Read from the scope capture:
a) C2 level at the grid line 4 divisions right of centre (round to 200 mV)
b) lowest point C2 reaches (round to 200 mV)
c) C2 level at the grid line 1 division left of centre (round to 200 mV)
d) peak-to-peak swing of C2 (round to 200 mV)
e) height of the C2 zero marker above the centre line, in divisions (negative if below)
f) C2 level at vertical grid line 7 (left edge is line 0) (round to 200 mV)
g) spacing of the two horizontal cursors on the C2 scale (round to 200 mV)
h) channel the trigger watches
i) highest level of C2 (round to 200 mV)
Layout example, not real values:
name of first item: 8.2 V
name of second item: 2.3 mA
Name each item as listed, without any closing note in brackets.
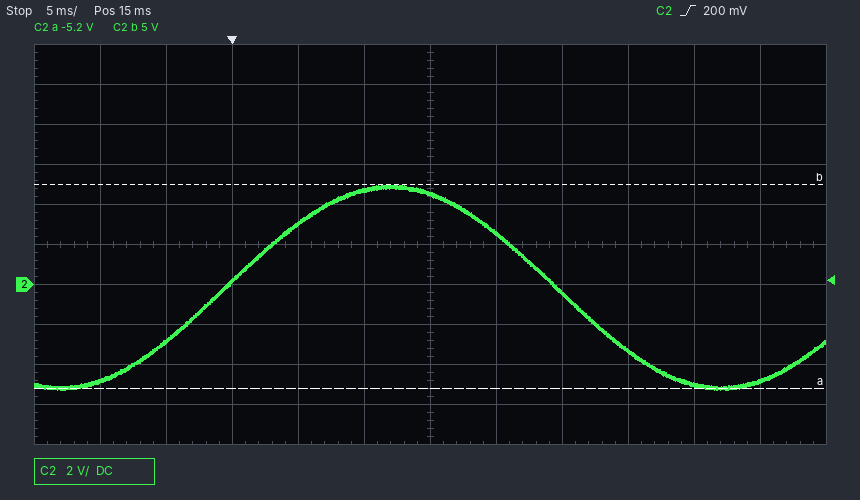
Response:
C2 level at the grid line 4 divisions right of centre: -5.0 V
lowest point C2 reaches: -5.2 V
C2 level at the grid line 1 division left of centre: 4.8 V
peak-to-peak swing of C2: 10.2 V
height of the C2 zero marker above the centre line, in divisions: -1.0 div
C2 level at vertical grid line 7 (left edge is line 0): 2.6 V
spacing of the two horizontal cursors on the C2 scale: 10.2 V
channel the trigger watches: C2
highest level of C2: 5.0 V
